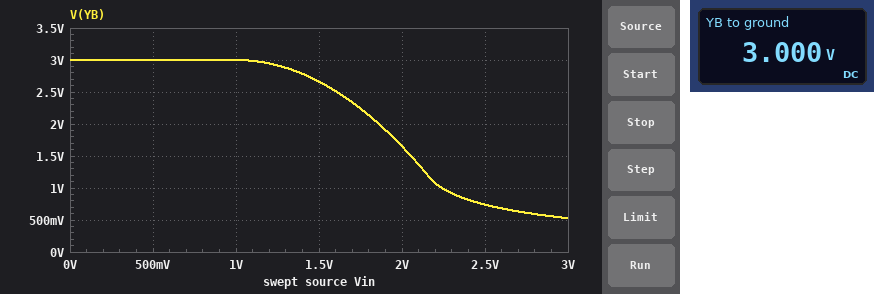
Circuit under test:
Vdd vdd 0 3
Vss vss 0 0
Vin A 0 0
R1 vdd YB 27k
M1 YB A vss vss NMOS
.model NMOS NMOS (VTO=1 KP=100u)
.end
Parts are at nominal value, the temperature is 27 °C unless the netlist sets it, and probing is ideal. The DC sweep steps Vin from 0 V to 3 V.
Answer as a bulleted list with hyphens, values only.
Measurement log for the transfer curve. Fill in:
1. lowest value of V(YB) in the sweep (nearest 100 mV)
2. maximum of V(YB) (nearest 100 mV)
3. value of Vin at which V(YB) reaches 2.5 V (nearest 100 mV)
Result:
- 500 mV
- 3.0 V
- 1.6 V
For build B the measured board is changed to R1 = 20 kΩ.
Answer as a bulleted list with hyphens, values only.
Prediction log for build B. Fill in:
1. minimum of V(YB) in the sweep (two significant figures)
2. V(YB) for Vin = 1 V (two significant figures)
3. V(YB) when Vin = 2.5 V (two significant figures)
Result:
- 700 mV
- 3.0 V
- 1.0 V
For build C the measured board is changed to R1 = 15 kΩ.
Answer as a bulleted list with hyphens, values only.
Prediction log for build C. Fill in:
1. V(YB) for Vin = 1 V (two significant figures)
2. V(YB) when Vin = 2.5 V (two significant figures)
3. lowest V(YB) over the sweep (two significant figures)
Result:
- 3.0 V
- 1.3 V
- 900 mV
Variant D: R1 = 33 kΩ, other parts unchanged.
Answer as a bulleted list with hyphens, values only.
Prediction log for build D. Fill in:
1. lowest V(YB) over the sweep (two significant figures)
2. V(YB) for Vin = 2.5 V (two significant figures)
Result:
- 440 mV
- 610 mV
